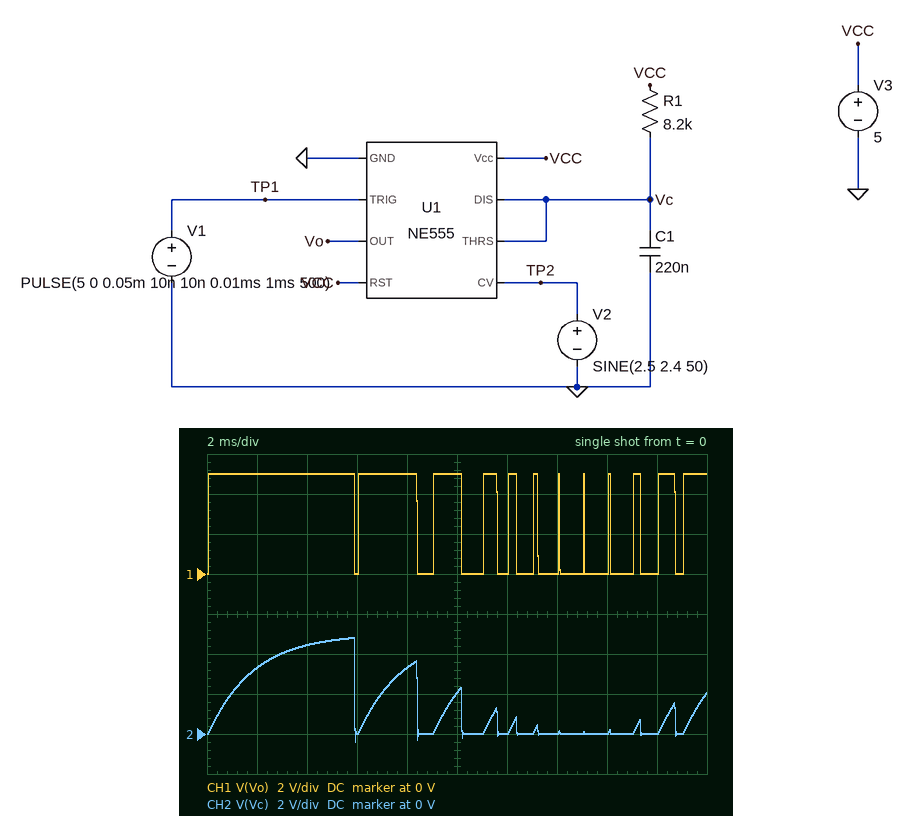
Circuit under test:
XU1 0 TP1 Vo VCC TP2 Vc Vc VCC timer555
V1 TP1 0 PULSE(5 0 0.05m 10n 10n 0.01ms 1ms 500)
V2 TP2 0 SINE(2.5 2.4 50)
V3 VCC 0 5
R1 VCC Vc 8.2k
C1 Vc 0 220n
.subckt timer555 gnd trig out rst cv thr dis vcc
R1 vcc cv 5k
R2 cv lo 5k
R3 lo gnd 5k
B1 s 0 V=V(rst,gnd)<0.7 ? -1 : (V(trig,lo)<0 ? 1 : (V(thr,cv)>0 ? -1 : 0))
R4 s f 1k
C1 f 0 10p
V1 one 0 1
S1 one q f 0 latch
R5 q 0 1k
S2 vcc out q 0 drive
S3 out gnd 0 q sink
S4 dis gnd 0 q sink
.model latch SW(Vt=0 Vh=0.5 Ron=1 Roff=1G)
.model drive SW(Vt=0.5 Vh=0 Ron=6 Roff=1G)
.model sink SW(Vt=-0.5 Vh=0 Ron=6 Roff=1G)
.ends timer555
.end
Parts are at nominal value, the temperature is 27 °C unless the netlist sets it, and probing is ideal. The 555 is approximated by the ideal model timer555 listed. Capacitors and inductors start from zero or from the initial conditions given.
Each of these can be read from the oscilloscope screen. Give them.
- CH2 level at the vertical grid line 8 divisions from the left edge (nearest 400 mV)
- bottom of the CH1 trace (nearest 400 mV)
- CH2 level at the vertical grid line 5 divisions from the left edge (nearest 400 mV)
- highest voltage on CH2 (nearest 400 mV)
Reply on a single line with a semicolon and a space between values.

0 V; 0 V; 2.0 V; 4.8 V
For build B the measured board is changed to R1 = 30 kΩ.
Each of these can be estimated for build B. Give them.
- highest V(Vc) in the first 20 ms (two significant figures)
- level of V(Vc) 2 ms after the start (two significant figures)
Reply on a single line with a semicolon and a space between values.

3.6 V; 1.3 V
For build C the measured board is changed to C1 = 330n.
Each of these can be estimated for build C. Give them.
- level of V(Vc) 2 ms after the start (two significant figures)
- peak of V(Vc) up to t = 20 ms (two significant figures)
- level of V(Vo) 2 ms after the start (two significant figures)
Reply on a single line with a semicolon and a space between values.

2.6 V; 4.6 V; 5.0 V
